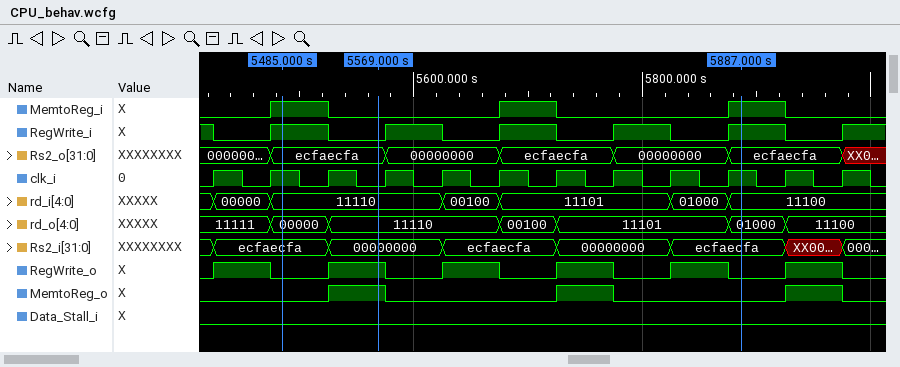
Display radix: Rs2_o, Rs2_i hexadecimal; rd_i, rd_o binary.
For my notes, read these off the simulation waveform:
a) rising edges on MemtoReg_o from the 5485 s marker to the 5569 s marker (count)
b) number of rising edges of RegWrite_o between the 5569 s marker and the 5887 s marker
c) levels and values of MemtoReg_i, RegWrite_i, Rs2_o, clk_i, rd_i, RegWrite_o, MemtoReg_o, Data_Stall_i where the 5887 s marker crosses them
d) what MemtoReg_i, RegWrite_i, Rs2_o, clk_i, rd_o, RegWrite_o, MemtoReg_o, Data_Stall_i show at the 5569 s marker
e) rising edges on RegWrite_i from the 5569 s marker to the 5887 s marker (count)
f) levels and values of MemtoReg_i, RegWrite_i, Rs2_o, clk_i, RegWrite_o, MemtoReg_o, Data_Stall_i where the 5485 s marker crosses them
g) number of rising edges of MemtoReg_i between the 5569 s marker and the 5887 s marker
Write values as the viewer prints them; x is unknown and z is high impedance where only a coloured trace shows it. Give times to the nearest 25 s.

1
3
MemtoReg_i=1, RegWrite_i=1, Rs2_o=ecfaecfa, clk_i=1, rd_i=11100, RegWrite_o=0, MemtoReg_o=0, Data_Stall_i=0
MemtoReg_i=0, RegWrite_i=0, Rs2_o=ecfaecfa, clk_i=0, rd_o=11110, RegWrite_o=1, MemtoReg_o=1, Data_Stall_i=0
4
MemtoReg_i=1, RegWrite_i=1, Rs2_o=ecfaecfa, clk_i=1, RegWrite_o=0, MemtoReg_o=0, Data_Stall_i=0
2
